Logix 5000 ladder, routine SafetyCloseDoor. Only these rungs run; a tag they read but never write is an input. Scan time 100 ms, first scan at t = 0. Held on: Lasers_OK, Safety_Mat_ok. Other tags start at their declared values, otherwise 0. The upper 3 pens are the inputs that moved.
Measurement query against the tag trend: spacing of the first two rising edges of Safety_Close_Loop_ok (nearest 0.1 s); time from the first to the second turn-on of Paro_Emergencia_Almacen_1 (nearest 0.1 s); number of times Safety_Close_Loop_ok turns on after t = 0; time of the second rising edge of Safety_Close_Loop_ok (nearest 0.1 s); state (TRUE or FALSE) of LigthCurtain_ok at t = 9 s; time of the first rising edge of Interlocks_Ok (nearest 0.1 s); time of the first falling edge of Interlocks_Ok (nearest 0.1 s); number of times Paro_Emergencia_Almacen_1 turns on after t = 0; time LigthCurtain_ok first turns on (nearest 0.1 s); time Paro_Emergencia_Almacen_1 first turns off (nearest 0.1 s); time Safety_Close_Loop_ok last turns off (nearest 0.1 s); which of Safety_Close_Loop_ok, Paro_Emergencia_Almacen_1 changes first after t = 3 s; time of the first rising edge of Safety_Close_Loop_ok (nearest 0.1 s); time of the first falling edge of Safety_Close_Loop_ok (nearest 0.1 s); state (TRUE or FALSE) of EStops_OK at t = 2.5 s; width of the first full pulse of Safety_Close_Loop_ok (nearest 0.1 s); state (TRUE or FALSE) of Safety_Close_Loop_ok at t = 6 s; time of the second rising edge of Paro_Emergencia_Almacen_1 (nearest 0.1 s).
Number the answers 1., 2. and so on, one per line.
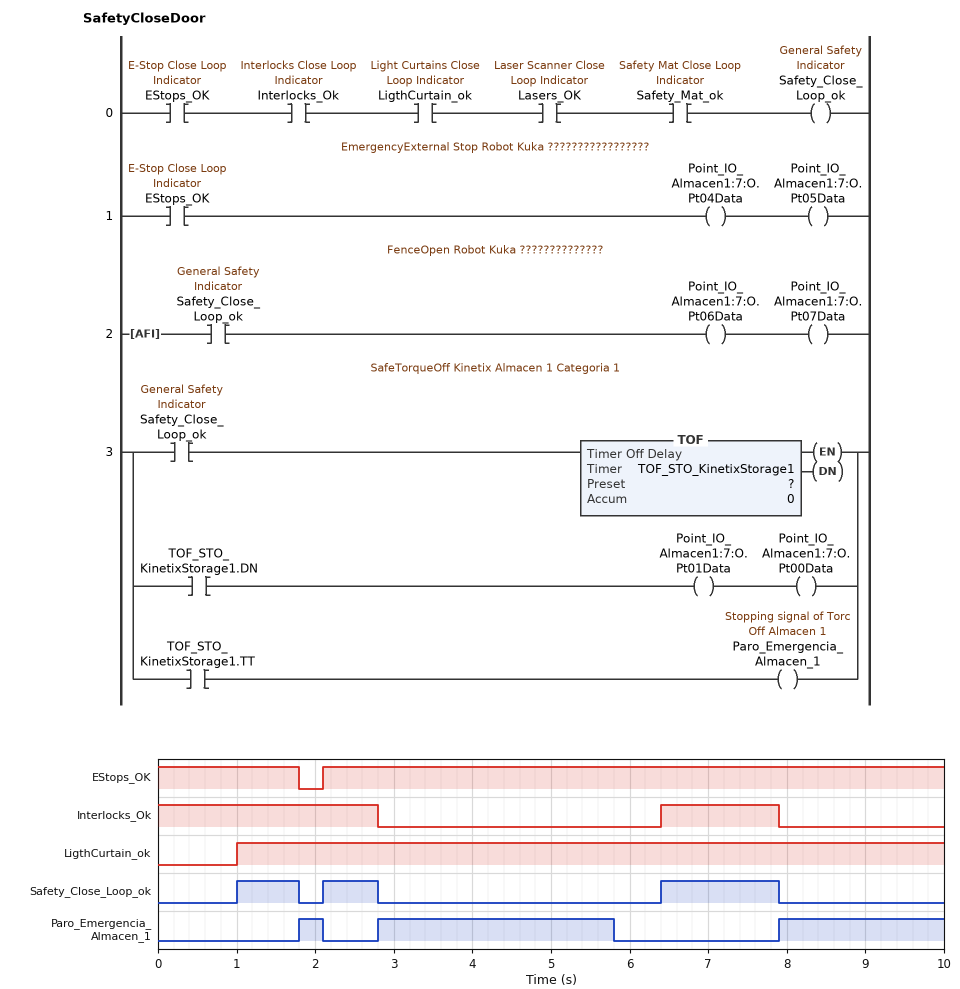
1. 1.1 s
2. 1.0 s
3. 3
4. 2.1 s
5. TRUE
6. 6.4 s
7. 2.8 s
8. 3
9. 1.0 s
10. 2.1 s
11. 7.9 s
12. Paro_Emergencia_Almacen_1
13. 1.0 s
14. 1.8 s
15. TRUE
16. 0.8 s
17. FALSE
18. 2.8 s
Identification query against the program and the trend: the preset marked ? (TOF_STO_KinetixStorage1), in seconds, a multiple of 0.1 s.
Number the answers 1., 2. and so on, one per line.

1. 3.0 s
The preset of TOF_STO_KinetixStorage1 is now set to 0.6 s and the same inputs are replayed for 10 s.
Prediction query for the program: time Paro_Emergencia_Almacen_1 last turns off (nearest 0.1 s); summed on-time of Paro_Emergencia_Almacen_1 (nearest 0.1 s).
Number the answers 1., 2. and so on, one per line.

1. 8.5 s
2. 1.5 s
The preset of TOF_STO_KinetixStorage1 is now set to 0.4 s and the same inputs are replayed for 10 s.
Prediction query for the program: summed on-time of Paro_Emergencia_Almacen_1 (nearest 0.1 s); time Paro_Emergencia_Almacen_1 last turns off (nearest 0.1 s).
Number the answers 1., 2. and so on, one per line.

1. 1.1 s
2. 8.3 s
